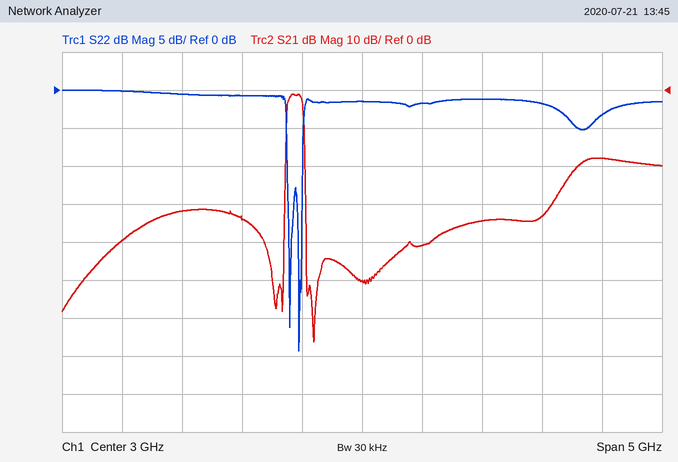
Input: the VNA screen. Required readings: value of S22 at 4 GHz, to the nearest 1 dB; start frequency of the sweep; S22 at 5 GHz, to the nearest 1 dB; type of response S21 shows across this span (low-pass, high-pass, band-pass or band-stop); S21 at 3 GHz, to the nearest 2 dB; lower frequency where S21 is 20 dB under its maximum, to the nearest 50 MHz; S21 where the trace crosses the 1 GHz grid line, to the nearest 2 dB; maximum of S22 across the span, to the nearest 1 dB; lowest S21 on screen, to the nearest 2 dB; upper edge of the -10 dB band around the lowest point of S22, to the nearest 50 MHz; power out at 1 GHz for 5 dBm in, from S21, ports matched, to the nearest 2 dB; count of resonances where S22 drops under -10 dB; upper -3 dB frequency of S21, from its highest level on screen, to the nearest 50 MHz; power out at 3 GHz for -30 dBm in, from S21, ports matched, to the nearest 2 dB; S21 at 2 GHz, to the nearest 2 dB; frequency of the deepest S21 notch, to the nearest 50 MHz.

-1 dB
500 MHz
-3 dB
band-pass
-50 dB
2.35 GHz
-40 dB
0 dB
-66 dB
2.50 GHz
-34 dBm
2
2.50 GHz
-80 dBm
-34 dB
2.60 GHz
